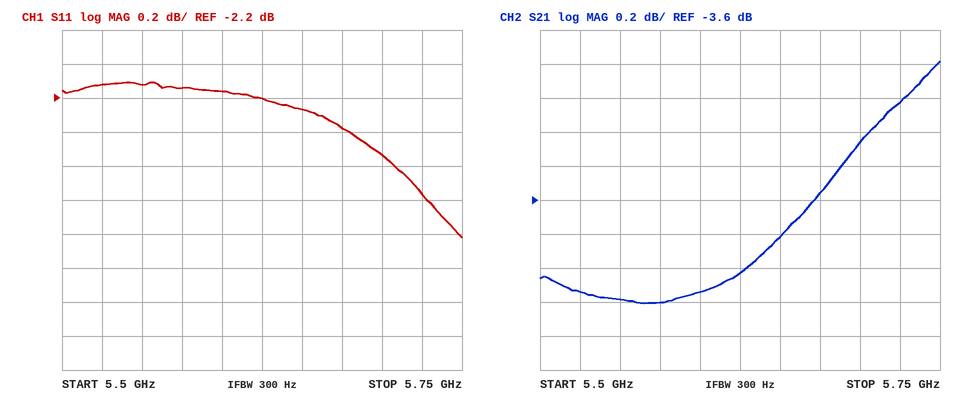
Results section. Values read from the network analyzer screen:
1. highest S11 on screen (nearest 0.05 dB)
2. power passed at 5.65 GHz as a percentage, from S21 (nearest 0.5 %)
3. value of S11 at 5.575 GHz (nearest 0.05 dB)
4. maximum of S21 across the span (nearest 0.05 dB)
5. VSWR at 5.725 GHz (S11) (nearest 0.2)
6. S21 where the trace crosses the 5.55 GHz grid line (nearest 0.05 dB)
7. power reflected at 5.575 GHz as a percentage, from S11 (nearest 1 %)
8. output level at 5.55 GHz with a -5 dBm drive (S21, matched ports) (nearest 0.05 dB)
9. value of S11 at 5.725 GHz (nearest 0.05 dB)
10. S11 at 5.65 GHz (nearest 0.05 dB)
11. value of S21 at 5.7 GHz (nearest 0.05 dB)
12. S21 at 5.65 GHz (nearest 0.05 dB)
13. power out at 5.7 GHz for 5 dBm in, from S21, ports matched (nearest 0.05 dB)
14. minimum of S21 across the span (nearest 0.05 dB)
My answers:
-2.10 dB
41.5 %
-2.15 dB
-2.80 dB
6.4
-4.20 dB
61 %
-9.20 dBm
-2.75 dB
-2.25 dB
-3.25 dB
-3.80 dB
1.75 dBm
-4.20 dB
